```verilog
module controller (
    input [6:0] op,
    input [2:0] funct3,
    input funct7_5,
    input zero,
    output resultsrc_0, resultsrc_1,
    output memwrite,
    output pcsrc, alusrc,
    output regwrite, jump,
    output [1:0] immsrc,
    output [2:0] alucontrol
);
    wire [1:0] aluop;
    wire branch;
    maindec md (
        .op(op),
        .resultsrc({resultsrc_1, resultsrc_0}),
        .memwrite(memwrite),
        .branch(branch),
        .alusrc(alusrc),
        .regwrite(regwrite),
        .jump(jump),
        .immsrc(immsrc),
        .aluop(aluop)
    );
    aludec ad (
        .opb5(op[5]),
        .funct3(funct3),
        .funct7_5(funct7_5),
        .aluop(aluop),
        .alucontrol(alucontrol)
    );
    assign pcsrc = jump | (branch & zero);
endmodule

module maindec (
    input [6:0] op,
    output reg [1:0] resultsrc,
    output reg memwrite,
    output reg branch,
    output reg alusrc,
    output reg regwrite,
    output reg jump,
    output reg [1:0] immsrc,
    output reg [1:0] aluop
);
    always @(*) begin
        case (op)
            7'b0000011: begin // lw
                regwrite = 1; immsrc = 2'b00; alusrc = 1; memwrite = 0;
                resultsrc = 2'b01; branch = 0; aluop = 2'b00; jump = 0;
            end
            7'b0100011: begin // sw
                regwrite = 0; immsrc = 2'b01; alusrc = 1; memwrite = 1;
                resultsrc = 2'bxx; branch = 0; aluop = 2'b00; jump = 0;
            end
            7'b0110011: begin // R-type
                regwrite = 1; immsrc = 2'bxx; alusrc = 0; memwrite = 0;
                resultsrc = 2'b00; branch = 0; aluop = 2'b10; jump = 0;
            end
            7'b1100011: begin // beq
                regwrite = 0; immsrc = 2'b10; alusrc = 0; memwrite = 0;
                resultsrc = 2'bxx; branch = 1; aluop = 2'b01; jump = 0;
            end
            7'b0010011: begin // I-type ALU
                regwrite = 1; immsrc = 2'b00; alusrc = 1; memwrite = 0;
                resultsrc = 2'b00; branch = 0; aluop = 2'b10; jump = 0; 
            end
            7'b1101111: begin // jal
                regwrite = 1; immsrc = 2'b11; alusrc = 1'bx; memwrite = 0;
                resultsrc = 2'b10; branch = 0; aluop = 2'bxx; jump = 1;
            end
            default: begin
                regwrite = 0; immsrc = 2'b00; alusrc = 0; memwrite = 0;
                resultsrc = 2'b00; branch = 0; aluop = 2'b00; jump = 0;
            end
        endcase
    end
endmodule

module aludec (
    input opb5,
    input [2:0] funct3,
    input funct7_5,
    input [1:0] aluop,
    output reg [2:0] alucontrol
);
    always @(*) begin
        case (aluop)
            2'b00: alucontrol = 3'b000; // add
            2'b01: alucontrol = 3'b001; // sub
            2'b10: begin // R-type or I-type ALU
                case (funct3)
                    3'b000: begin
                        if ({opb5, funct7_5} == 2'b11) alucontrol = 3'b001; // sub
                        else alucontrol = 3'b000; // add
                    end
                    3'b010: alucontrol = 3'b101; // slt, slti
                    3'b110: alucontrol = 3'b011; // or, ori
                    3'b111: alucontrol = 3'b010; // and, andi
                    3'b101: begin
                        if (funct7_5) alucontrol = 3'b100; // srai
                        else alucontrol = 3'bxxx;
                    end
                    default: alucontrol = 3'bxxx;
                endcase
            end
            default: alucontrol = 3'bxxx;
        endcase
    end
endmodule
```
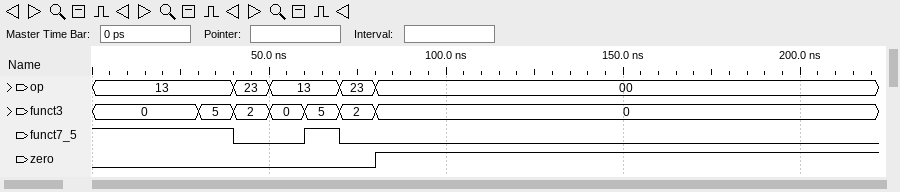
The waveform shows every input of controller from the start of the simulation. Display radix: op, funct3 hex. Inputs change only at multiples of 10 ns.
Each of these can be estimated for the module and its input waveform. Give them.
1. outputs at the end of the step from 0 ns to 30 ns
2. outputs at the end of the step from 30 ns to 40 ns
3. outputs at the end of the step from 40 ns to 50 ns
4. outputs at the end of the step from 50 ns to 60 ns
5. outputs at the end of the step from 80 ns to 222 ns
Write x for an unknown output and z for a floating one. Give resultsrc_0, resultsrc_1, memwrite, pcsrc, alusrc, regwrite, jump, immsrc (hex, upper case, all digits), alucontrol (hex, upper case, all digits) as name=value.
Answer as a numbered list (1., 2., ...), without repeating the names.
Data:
1. resultsrc_0=0, resultsrc_1=0, memwrite=0, pcsrc=0, alusrc=1, regwrite=1, jump=0, immsrc=0, alucontrol=0
2. resultsrc_0=0, resultsrc_1=0, memwrite=0, pcsrc=0, alusrc=1, regwrite=1, jump=0, immsrc=0, alucontrol=4
3. resultsrc_0=x, resultsrc_1=x, memwrite=1, pcsrc=0, alusrc=1, regwrite=0, jump=0, immsrc=1, alucontrol=0
4. resultsrc_0=0, resultsrc_1=0, memwrite=0, pcsrc=0, alusrc=1, regwrite=1, jump=0, immsrc=0, alucontrol=0
5. resultsrc_0=0, resultsrc_1=0, memwrite=0, pcsrc=0, alusrc=0, regwrite=0, jump=0, immsrc=0, alucontrol=0
